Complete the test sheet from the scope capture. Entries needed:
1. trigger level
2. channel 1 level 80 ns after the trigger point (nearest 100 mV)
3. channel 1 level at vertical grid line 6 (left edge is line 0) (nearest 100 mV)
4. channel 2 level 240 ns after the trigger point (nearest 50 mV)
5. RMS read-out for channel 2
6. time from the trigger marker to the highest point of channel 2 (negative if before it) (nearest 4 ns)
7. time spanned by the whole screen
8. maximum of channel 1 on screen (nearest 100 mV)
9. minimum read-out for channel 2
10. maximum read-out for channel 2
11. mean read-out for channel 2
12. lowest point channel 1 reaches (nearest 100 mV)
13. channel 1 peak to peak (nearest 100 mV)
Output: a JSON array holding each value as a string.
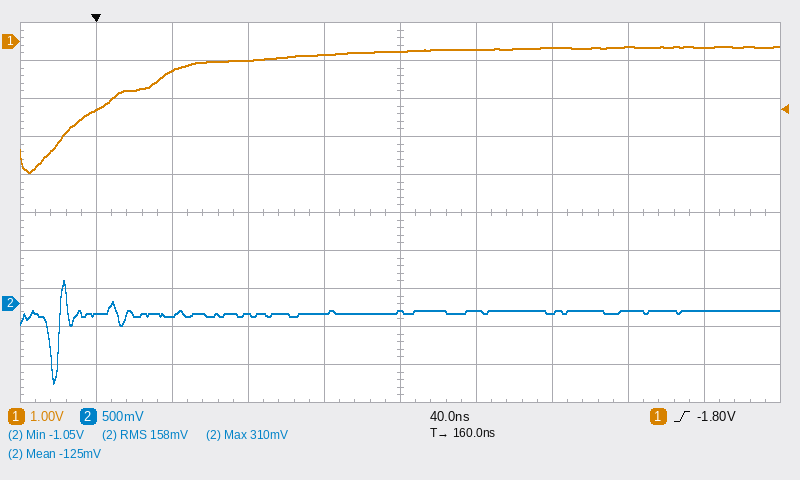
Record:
["-1.80 V", "-500 mV", "-200 mV", "-100 mV", "158 mV", "-16 ns", "400 ns", "-100 mV", "-1.05 V", "310 mV", "-125 mV", "-3.4 V", "3.3 V"]
